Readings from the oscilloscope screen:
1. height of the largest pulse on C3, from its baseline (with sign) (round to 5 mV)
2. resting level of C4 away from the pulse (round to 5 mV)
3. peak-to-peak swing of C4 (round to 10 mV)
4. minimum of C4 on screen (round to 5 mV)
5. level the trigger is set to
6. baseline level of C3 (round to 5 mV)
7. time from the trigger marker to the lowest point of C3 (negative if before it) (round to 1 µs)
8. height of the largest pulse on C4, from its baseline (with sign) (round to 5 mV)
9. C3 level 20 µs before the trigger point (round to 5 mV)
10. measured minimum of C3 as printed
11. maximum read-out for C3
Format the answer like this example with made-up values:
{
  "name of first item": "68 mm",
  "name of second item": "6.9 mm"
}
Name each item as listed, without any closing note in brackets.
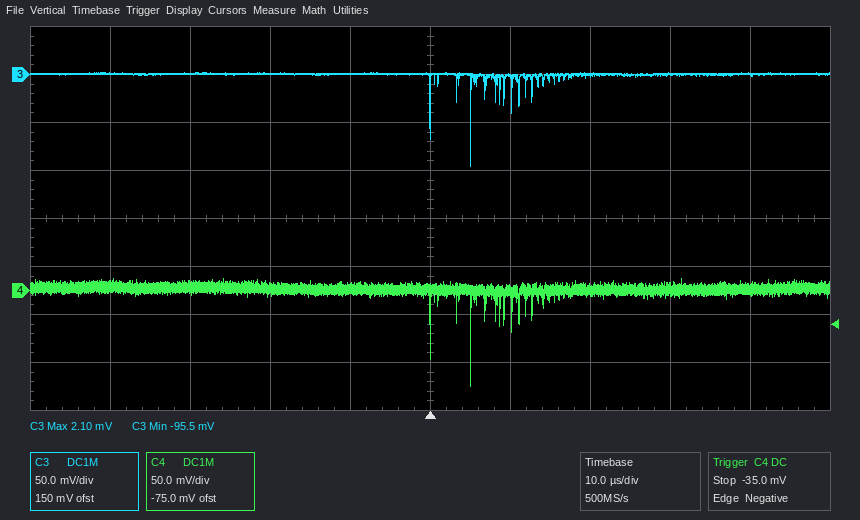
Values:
{
  "height of the largest pulse on C3, from its baseline (with sign)": "-95 mV",
  "resting level of C4 away from the pulse": "0 mV",
  "peak-to-peak swing of C4": "110 mV",
  "minimum of C4 on screen": "-100 mV",
  "level the trigger is set to": "-35.0 mV",
  "baseline level of C3": "0 mV",
  "time from the trigger marker to the lowest point of C3 (negative if before it)": "+5 µs",
  "height of the largest pulse on C4, from its baseline (with sign)": "-100 mV",
  "C3 level 20 µs before the trigger point": "0 mV",
  "measured minimum of C3 as printed": "-95.5 mV",
  "maximum read-out for C3": "2.10 mV"
}
